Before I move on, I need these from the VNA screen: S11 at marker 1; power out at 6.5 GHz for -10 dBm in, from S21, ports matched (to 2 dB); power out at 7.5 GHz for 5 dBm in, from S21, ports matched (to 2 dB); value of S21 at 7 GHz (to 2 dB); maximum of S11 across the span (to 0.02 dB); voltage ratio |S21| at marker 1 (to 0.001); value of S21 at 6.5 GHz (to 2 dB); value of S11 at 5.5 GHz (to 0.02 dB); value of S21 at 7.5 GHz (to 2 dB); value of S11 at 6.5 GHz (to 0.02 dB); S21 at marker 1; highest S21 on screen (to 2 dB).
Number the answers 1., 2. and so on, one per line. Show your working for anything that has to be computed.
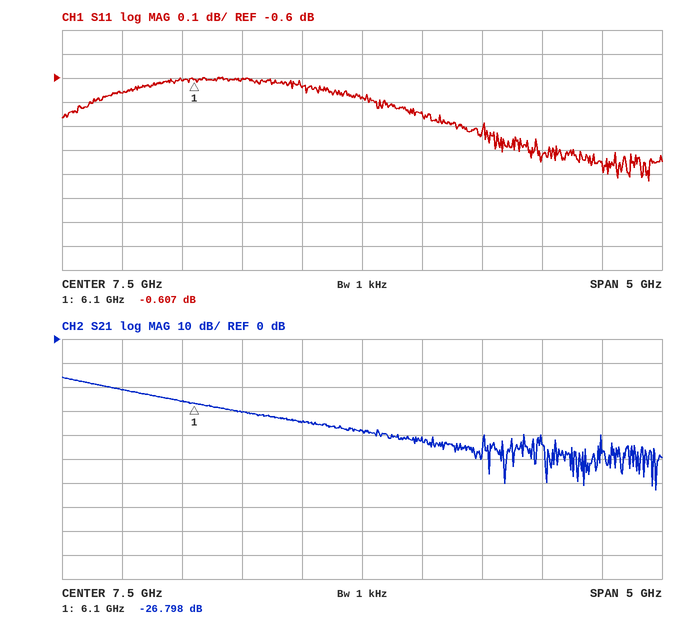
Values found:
1. -0.607 dB
2. -10 dBm + (-30 dB) = -40 dBm
3. 5 dBm + (-38 dB) = -34 dBm
4. -34 dB
5. -0.60 dB
6. 10^(-26.798/20) ≈ 0.046
7. -30 dB
8. -0.66 dB
9. -38 dB
10. -0.60 dB
11. -26.798 dB
12. -16 dB
